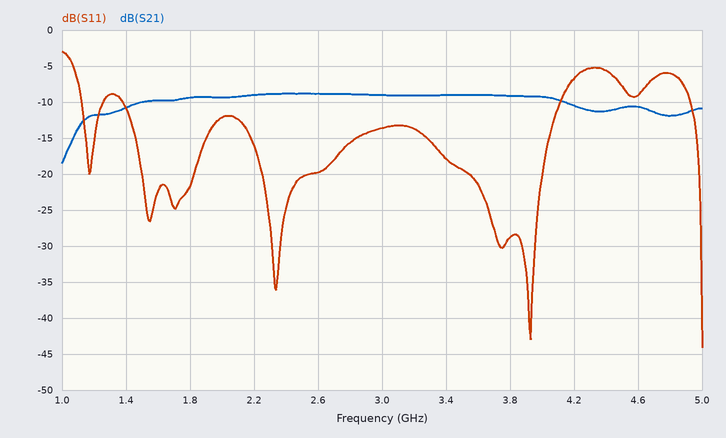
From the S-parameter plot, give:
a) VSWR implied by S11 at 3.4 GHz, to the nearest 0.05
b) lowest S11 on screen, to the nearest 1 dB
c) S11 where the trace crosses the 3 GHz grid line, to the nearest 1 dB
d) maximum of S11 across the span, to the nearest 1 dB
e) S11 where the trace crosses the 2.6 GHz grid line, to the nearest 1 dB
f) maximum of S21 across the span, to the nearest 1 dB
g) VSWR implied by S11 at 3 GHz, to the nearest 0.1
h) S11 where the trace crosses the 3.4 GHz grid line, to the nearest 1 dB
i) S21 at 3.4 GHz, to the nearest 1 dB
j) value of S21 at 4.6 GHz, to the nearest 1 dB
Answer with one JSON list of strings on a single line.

["1.30", "-44 dB", "-14 dB", "-3 dB", "-20 dB", "-9 dB", "1.5", "-18 dB", "-9 dB", "-11 dB"]
